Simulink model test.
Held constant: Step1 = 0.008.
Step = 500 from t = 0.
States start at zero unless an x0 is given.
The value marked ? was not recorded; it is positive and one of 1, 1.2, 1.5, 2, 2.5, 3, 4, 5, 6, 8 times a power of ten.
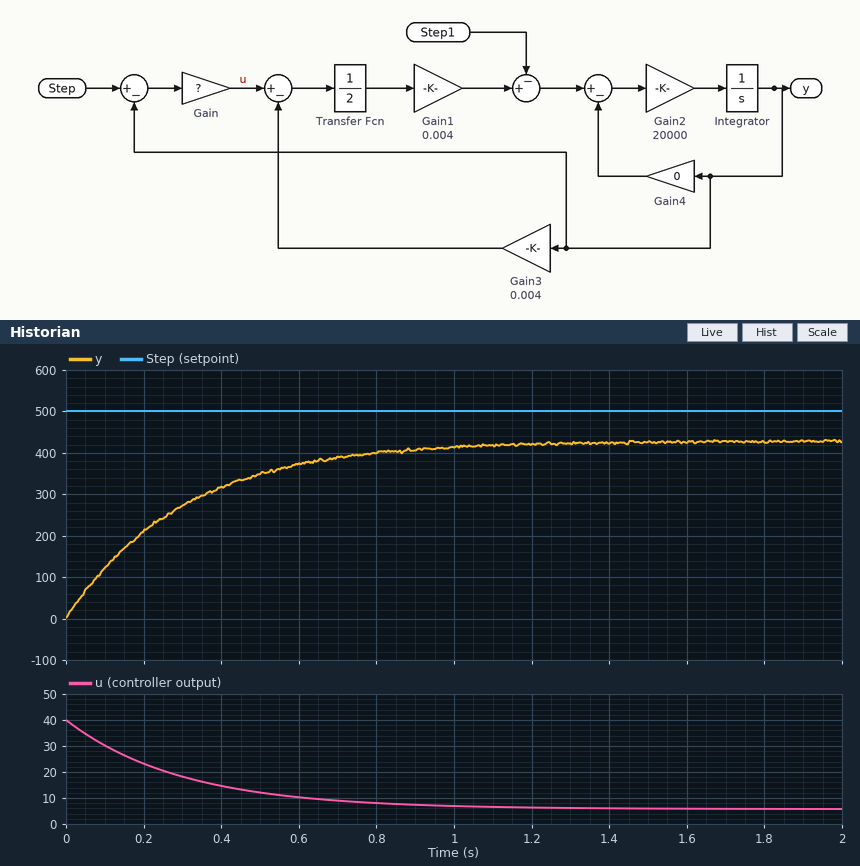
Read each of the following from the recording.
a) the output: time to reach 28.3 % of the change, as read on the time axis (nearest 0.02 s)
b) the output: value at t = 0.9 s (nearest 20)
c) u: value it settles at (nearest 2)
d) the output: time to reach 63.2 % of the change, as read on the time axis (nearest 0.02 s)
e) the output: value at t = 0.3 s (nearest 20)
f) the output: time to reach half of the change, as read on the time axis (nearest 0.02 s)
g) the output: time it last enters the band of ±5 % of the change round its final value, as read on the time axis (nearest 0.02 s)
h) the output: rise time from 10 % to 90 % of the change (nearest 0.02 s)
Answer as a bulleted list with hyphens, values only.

- 0.10 s
- 400
- 6
- 0.30 s
- 280
- 0.20 s
- 0.90 s
- 0.66 s
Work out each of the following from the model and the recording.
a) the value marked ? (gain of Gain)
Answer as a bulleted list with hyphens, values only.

- 0.08
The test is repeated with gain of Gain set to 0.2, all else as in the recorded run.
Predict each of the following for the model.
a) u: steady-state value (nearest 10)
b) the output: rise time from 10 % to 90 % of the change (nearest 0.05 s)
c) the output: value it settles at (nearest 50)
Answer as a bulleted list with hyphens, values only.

- 10
- 0.25 s
- 450
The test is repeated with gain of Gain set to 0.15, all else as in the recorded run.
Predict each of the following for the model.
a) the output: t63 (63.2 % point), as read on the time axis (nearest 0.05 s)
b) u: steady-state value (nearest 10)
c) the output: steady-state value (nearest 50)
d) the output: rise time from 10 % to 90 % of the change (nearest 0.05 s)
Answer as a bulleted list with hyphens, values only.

- 0.15 s
- 10
- 450
- 0.35 s
